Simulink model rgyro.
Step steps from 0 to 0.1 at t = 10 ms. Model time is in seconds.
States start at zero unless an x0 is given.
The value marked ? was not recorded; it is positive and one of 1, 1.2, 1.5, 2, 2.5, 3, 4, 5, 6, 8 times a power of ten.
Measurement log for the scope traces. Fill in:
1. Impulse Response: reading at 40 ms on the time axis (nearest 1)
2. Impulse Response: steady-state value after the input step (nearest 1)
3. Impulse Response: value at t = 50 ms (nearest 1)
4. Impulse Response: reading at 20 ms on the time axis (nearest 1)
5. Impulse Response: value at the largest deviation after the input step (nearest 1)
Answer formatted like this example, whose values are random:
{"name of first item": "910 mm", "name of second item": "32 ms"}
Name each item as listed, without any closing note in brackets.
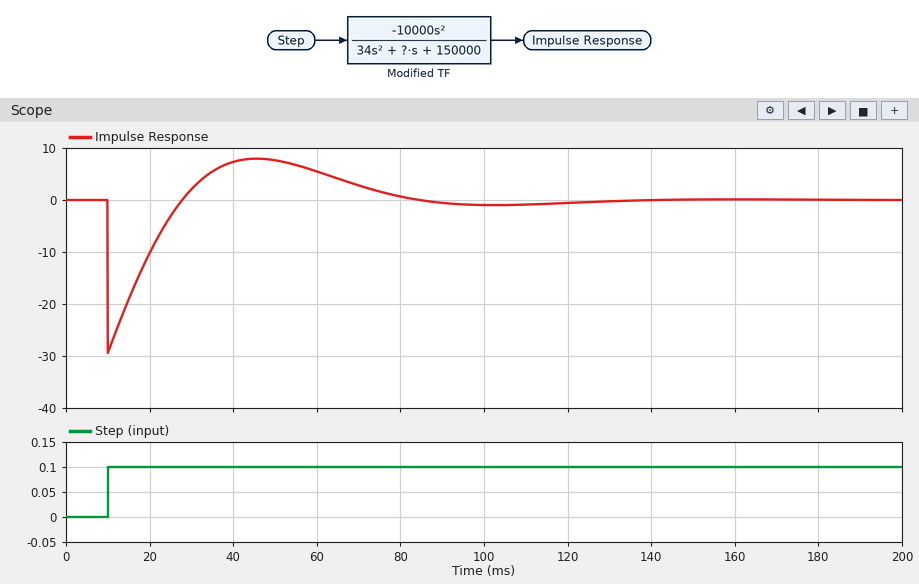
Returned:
{"Impulse Response: reading at 40 ms on the time axis": "7", "Impulse Response: steady-state value after the input step": "0", "Impulse Response: value at t = 50 ms": "8", "Impulse Response: reading at 20 ms on the time axis": "-10", "Impulse Response: value at the largest deviation after the input step": "-29"}
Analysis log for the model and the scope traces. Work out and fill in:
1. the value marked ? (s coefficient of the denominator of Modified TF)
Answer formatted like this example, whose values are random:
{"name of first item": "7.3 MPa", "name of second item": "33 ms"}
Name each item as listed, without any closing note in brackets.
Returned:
{"the value marked ?": "2500"}
